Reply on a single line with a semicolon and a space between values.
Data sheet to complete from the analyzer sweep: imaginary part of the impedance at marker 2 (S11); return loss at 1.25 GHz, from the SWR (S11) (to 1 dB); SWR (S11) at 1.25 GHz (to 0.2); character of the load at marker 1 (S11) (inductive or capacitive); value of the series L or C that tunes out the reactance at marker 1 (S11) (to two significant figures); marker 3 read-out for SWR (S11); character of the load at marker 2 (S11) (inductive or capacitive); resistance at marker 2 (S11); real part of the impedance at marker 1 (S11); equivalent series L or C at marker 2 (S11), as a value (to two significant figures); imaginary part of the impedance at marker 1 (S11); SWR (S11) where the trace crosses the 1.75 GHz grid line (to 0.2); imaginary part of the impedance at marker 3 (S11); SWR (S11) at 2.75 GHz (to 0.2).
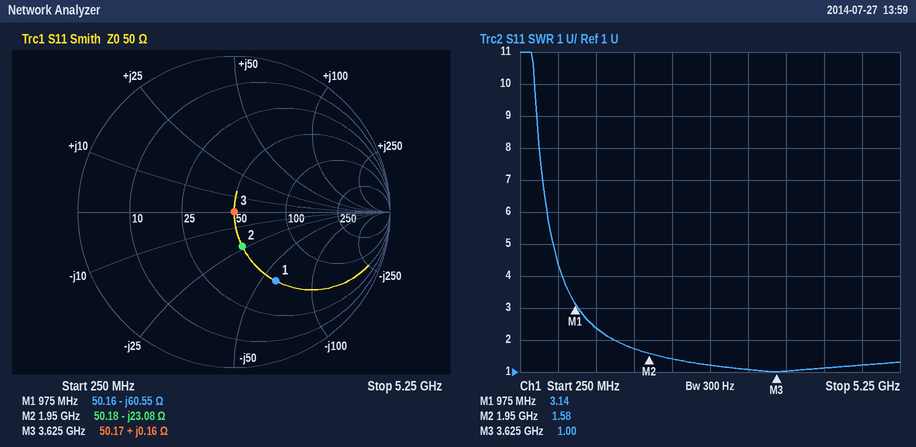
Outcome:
-23.08 Ω; 8 dB; 2.4; capacitive; 9.9 nH; 1.00; capacitive; 50.18 Ω; 50.16 Ω; 3.5 pF; -60.55 Ω; 1.8; +0.16 Ω; 1.2
